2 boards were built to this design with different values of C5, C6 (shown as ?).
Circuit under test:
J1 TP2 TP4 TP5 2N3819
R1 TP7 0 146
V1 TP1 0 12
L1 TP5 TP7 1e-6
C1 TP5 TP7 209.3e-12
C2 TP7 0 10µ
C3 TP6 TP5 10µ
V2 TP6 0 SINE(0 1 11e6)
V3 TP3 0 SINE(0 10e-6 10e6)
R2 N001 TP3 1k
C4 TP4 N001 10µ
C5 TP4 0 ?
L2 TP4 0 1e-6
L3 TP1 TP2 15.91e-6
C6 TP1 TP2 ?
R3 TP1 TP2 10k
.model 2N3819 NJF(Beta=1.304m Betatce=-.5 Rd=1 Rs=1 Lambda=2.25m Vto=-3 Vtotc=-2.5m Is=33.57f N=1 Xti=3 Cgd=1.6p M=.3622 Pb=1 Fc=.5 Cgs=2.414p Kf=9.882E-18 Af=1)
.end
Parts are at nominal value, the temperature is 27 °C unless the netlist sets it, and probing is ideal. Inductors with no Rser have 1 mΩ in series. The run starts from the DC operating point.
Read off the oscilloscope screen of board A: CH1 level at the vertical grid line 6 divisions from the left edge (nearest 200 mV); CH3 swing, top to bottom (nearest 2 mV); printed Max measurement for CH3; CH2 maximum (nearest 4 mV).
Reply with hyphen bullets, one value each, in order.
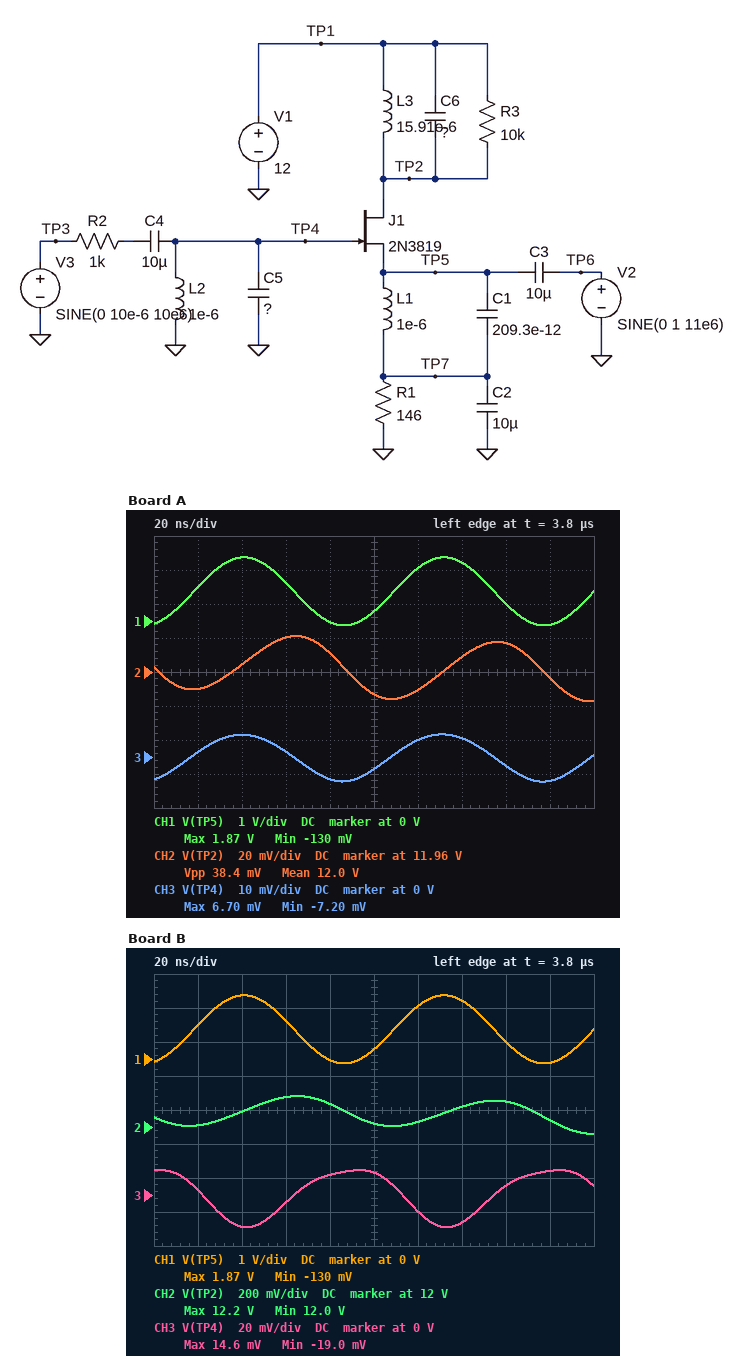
- 1.6 V
- 14 mV
- 6.70 mV
- 11.980 V
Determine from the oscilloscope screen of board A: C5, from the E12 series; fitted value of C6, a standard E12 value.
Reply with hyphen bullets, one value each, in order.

- 470 pF
- 4.7 nF
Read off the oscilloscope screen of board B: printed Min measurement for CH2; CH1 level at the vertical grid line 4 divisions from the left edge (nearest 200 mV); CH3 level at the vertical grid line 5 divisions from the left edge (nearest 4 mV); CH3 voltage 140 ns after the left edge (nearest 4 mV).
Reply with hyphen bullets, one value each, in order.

- 12.0 V
- 0 V
- 12 mV
- -16 mV
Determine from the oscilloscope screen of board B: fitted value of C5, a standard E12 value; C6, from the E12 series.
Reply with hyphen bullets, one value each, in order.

- 100 pF
- 1 nF
